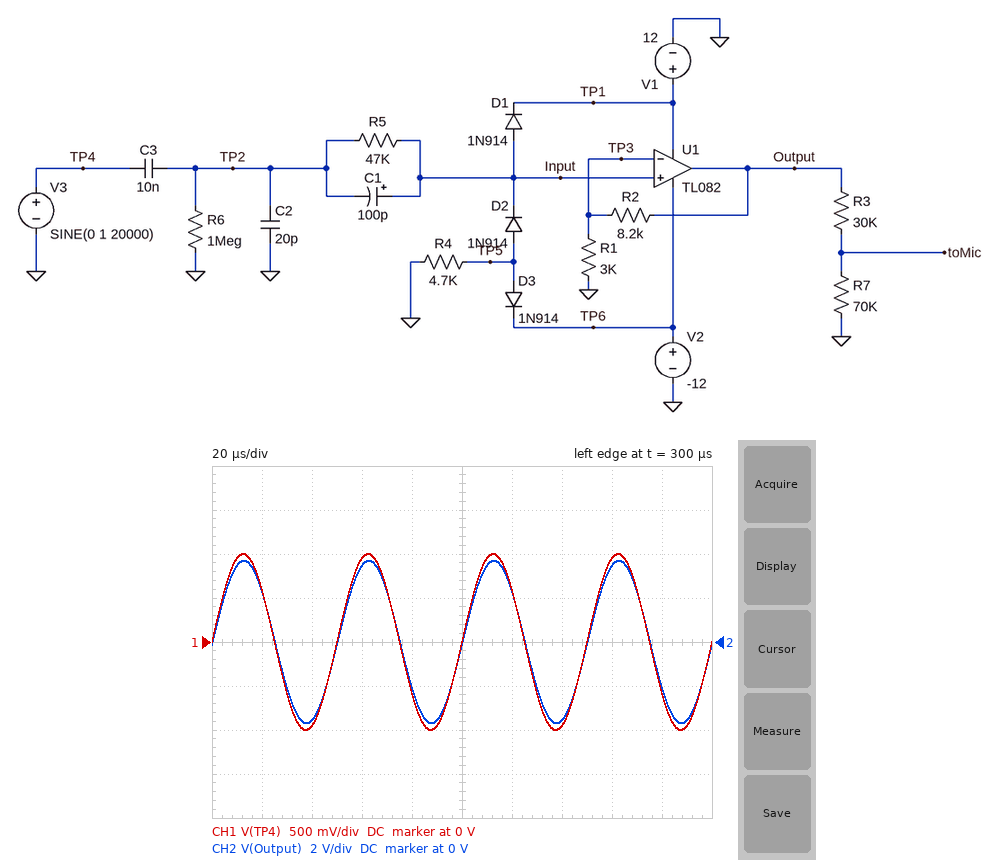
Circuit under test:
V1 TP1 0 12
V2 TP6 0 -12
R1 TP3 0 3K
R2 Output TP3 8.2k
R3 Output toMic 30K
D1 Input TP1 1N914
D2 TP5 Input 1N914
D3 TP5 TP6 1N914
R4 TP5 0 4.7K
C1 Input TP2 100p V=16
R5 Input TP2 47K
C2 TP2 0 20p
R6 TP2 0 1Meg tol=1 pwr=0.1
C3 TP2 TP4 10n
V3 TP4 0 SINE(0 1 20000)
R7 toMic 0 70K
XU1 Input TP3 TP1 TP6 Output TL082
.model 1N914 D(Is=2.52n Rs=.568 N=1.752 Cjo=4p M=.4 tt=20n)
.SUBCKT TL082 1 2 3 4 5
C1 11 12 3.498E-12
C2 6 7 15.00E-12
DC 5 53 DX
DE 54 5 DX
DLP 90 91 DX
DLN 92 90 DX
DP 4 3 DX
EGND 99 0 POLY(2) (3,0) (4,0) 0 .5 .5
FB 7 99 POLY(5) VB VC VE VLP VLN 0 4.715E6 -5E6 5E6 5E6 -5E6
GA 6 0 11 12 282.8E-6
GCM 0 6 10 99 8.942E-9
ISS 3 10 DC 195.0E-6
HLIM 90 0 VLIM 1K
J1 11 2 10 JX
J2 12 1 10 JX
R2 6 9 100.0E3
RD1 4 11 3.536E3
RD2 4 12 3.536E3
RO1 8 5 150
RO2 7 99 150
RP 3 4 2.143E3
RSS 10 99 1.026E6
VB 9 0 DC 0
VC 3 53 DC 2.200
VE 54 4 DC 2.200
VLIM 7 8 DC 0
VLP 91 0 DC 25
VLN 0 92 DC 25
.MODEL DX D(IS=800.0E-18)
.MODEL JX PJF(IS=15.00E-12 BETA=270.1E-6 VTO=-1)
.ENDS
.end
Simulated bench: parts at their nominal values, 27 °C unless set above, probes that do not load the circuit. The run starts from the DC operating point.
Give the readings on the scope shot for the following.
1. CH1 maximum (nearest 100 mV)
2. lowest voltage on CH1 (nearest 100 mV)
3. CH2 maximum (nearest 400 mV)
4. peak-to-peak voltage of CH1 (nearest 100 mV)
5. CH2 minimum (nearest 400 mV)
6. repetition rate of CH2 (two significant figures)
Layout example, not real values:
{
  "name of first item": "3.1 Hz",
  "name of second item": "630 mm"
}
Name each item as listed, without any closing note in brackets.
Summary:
{
  "CH1 maximum": "1.0 V",
  "lowest voltage on CH1": "-1.0 V",
  "CH2 maximum": "3.6 V",
  "peak-to-peak voltage of CH1": "2.0 V",
  "CH2 minimum": "-3.6 V",
  "repetition rate of CH2": "20 kHz"
}
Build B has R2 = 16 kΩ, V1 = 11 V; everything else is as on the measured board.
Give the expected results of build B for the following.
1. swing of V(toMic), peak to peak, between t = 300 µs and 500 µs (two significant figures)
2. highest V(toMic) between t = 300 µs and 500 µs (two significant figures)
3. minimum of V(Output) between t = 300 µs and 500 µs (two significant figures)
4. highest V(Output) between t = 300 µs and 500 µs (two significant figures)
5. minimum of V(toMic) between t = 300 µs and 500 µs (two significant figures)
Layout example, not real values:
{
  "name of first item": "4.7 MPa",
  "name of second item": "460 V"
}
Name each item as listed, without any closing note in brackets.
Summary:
{
  "swing of V(toMic), peak to peak, between t = 300 µs and 500 µs": "8.8 V",
  "highest V(toMic) between t = 300 µs and 500 µs": "4.4 V",
  "minimum of V(Output) between t = 300 µs and 500 µs": "-6.3 V",
  "highest V(Output) between t = 300 µs and 500 µs": "6.3 V",
  "minimum of V(toMic) between t = 300 µs and 500 µs": "-4.4 V"
}
